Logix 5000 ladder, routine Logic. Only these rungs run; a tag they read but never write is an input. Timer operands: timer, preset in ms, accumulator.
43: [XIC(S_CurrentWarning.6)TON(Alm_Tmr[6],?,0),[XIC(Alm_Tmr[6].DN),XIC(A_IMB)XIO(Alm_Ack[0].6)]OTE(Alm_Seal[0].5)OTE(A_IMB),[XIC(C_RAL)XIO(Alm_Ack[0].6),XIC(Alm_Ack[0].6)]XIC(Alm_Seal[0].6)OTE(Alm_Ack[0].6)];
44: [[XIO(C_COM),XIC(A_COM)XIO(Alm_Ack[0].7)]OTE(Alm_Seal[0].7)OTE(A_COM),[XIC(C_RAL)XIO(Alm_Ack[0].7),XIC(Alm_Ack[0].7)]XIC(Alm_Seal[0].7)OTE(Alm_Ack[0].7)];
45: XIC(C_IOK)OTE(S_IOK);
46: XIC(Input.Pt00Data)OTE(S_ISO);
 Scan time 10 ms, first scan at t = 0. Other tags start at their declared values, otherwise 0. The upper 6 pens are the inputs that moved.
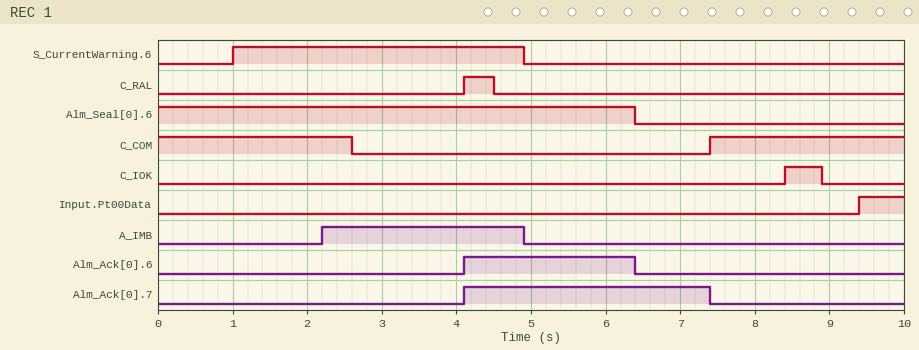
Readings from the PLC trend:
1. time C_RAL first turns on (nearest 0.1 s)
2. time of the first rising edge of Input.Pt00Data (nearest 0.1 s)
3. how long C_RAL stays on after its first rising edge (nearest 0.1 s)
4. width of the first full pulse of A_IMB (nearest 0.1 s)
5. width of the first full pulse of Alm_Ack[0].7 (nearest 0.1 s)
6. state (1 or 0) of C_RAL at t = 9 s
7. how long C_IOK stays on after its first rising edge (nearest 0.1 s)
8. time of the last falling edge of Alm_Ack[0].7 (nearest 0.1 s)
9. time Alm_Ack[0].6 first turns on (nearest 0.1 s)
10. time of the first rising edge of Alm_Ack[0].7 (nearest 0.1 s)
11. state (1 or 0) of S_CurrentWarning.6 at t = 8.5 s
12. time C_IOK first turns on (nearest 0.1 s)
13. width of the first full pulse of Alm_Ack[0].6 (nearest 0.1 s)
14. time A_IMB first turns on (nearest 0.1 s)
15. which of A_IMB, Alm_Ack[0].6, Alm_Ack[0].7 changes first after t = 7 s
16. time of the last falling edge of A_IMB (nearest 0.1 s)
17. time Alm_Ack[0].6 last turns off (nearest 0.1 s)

4.1 s
9.4 s
0.4 s
2.7 s
3.3 s
0
0.5 s
7.4 s
4.1 s
4.1 s
0
8.4 s
2.3 s
2.2 s
Alm_Ack[0].7
4.9 s
6.4 s
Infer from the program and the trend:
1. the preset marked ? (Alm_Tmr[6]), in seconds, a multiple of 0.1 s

1.2 s
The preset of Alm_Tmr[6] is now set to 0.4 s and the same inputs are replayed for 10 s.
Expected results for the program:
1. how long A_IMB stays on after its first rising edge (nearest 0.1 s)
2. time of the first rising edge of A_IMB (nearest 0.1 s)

3.5 s
1.4 s
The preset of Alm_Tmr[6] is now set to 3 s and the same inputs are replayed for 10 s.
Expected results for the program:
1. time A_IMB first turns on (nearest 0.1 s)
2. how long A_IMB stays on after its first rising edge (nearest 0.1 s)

4.0 s
0.9 s
